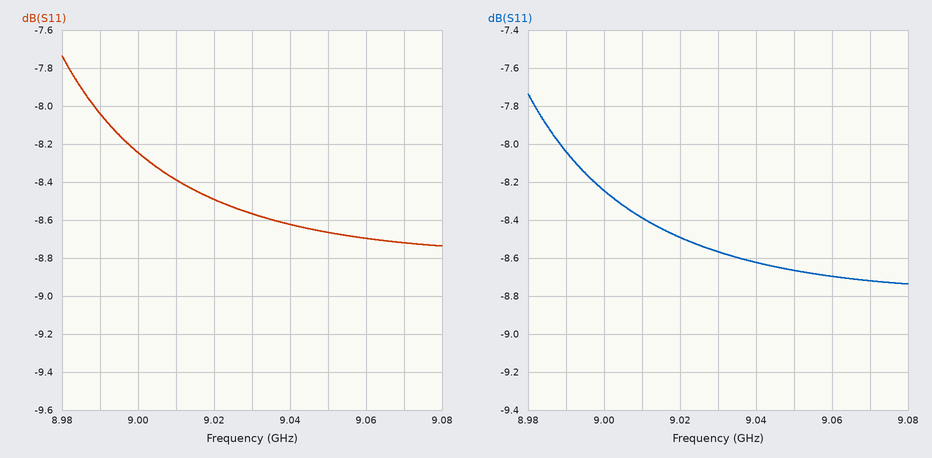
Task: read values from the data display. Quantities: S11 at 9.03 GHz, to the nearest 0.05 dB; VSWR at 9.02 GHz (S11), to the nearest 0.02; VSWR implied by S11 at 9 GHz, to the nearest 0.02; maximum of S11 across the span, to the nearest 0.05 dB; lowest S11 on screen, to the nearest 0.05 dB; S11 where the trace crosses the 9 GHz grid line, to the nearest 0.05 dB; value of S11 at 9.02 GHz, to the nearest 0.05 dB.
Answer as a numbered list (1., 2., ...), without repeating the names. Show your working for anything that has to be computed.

1. -8.55 dB
2. |Γ| = 10^(-8.5/20) = 0.3758; VSWR = (1 + 0.3758)/(1 − 0.3758) ≈ 2.20
3. |Γ| = 10^(-8.25/20) = 0.3868; VSWR = (1 + 0.3868)/(1 − 0.3868) ≈ 2.26
4. -7.75 dB
5. -8.75 dB
6. -8.25 dB
7. -8.50 dB
